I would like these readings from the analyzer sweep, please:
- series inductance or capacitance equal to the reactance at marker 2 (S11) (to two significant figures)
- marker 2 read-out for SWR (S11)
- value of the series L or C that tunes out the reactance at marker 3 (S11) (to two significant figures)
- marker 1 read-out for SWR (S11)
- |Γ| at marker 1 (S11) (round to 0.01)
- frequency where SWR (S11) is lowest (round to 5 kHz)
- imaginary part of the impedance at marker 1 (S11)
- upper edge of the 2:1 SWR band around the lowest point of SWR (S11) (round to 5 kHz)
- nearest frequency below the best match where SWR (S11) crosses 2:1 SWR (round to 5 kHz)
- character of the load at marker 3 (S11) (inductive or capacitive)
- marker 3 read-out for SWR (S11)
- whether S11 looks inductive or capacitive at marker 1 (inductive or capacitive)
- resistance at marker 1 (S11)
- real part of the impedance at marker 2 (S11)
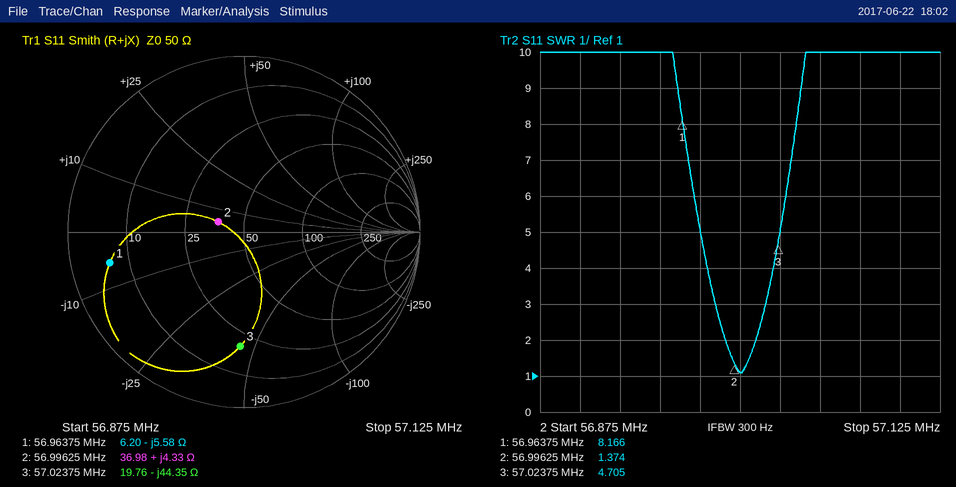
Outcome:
12 nH
1.374
120 nH
8.166
0.78
57.000 MHz
-5.58 Ω
57.010 MHz
56.990 MHz
capacitive
4.705
capacitive
6.20 Ω
36.98 Ω
